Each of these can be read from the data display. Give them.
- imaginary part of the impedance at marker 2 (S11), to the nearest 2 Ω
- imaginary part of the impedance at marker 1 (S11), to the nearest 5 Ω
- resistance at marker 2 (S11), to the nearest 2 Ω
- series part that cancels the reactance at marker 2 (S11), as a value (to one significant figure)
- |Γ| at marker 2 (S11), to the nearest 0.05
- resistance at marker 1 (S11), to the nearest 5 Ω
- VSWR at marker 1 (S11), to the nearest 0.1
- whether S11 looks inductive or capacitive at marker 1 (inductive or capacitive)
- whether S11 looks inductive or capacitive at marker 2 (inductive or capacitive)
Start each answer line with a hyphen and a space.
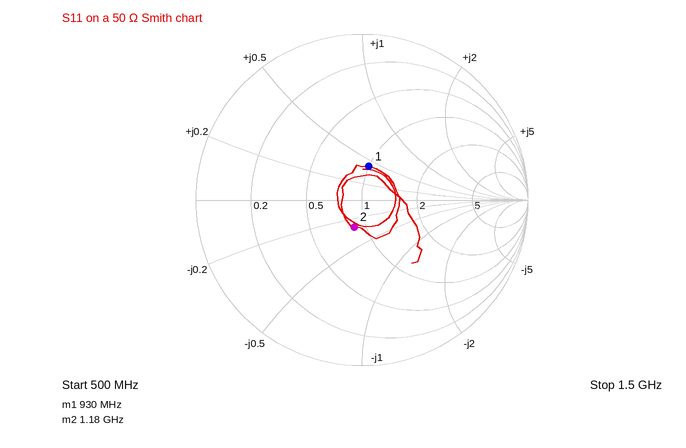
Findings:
- -14 Ω
- +20 Ω
- 44 Ω
- 2 nH
- 0.15
- 50 Ω
- 1.5
- inductive
- capacitive
